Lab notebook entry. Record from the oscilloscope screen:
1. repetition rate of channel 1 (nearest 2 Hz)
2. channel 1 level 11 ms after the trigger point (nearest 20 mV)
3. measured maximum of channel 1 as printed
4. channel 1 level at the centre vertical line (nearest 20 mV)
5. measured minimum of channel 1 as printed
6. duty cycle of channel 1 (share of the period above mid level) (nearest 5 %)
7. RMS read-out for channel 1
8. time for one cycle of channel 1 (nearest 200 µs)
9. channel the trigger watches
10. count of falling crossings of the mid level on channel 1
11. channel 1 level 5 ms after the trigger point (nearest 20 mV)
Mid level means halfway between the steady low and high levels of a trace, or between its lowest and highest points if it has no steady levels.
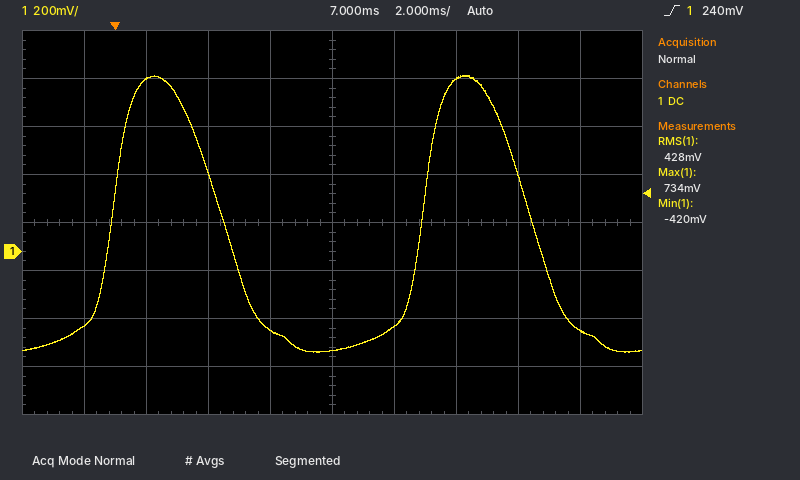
100 Hz
720 mV
734 mV
-420 mV
-420 mV
35 %
428 mV
10.0 ms
channel 1
2
-320 mV
